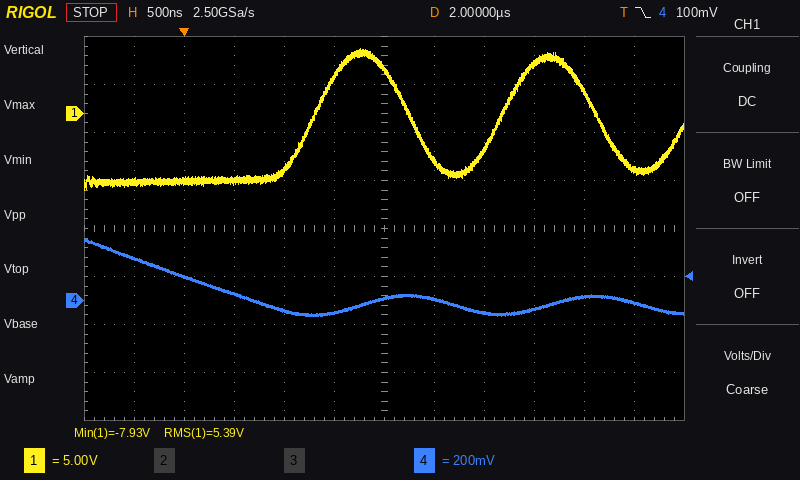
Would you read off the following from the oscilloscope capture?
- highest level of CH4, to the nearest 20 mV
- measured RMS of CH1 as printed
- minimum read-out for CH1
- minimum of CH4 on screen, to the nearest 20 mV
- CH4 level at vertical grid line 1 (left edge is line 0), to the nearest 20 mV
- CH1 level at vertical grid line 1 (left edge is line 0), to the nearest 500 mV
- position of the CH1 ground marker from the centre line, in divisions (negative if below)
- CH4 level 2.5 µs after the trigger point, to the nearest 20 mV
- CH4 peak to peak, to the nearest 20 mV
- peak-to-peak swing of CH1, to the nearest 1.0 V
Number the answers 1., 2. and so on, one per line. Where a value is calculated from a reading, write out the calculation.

1. 260 mV
2. 5.39 V
3. -7.93 V
4. -60 mV
5. 180 mV
6. -7.0 V
7. +2.4 div
8. 0 mV
9. 260 mV − (-60 mV) = 320 mV
10. 15.0 V
